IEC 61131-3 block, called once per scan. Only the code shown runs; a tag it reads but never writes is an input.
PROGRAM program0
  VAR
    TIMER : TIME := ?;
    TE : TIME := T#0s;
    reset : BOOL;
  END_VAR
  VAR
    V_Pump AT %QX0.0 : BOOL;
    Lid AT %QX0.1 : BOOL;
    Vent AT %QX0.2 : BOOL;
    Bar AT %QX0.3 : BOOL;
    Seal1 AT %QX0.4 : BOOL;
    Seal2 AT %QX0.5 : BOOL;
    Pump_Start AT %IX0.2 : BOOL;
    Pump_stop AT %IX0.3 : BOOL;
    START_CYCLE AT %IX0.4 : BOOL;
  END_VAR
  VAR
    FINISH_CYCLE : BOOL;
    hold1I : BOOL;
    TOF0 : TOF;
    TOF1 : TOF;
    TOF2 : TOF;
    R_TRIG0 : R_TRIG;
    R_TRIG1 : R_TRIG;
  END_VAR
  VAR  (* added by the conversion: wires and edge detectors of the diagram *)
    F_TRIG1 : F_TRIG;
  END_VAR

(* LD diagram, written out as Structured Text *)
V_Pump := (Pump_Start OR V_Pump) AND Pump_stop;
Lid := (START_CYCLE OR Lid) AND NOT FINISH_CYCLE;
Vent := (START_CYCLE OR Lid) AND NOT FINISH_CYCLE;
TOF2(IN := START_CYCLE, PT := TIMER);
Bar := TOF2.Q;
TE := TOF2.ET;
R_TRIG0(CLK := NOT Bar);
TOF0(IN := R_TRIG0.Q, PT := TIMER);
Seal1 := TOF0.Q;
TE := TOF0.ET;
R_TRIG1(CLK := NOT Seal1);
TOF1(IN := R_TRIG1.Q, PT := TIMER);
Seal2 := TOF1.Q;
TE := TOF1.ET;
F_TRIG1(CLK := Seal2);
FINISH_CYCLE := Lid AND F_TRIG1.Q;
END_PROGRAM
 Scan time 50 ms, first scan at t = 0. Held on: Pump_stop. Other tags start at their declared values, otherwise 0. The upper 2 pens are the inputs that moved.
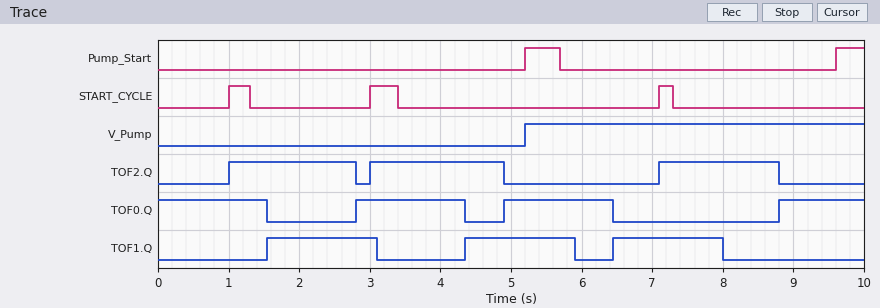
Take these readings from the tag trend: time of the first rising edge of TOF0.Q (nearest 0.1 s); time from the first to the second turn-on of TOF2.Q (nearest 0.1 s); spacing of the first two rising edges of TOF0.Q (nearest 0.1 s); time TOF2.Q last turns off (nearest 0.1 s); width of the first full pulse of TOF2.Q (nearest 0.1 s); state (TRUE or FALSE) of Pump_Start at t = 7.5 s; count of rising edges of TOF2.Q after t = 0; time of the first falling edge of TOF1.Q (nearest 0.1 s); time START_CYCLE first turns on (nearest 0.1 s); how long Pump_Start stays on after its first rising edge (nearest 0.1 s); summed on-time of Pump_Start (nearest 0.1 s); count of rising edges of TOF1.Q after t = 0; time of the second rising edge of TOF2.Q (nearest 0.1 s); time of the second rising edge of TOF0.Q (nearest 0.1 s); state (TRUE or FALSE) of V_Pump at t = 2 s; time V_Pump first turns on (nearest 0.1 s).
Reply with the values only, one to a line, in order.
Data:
2.8 s
2.0 s
2.1 s
8.8 s
1.8 s
FALSE
3
3.1 s
1.0 s
0.5 s
0.9 s
3
3.0 s
4.9 s
FALSE
5.2 s
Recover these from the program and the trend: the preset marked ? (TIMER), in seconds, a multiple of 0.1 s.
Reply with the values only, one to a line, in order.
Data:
1.5 s
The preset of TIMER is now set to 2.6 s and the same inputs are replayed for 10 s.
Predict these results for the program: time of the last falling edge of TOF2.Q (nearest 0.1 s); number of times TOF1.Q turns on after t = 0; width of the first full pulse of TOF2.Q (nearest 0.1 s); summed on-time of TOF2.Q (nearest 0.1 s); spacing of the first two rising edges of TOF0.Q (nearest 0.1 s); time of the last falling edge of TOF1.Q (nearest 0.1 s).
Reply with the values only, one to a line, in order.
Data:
9.9 s
2
5.0 s
7.8 s
3.9 s
5.3 s
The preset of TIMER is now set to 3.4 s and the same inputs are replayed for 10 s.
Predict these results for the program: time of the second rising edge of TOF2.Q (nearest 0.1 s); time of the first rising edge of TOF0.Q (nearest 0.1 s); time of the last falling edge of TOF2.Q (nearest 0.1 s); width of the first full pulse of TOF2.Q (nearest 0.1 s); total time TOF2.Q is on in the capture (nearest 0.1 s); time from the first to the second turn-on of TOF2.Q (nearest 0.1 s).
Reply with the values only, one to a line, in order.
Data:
7.1 s
6.8 s
6.8 s
5.8 s
8.7 s
6.1 s
